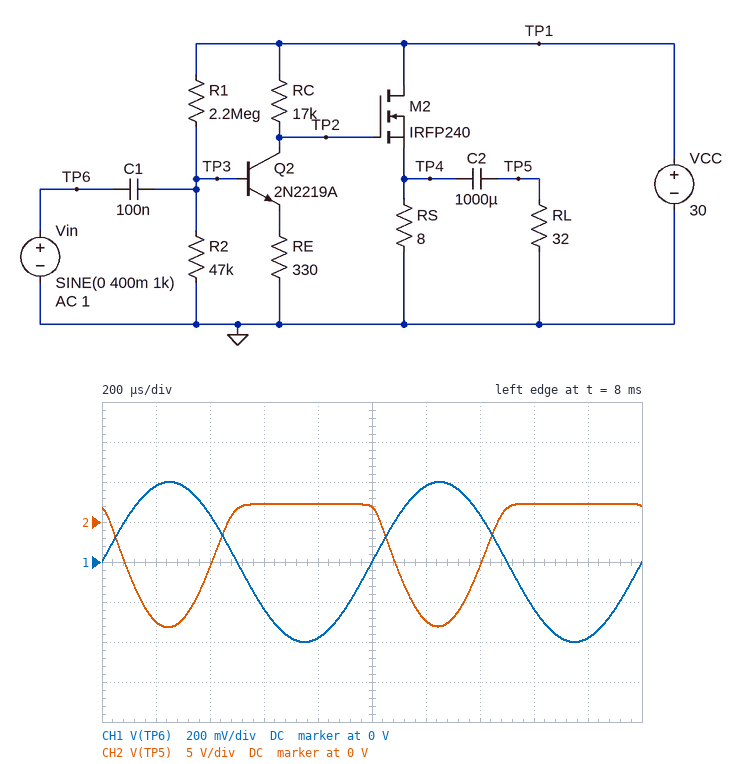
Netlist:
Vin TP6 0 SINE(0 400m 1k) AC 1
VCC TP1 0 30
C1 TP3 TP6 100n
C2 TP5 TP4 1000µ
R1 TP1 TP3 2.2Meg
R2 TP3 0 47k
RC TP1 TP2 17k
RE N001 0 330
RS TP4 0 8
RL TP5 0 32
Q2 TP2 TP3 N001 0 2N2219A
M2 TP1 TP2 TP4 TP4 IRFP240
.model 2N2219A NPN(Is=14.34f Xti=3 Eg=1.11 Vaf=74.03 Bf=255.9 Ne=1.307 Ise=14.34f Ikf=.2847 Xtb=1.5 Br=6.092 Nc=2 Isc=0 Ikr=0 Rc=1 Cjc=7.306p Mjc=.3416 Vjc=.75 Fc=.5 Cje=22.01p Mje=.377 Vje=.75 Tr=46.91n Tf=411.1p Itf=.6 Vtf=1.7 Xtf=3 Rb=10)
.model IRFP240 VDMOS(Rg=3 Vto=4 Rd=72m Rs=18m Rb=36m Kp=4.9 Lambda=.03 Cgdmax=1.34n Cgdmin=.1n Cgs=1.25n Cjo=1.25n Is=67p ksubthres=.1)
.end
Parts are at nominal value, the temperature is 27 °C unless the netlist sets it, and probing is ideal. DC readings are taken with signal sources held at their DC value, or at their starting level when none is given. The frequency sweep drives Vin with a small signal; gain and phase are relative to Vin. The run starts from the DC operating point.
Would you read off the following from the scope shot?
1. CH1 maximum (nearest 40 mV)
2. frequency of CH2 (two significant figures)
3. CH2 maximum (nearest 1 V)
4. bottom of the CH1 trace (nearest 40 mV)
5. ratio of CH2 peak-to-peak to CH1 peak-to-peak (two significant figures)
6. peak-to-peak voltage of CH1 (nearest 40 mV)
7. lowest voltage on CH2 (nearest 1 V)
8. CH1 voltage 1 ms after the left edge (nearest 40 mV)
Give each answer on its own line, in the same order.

400 mV
1.0 kHz
2 V
-400 mV
19
800 mV
-13 V
0 V
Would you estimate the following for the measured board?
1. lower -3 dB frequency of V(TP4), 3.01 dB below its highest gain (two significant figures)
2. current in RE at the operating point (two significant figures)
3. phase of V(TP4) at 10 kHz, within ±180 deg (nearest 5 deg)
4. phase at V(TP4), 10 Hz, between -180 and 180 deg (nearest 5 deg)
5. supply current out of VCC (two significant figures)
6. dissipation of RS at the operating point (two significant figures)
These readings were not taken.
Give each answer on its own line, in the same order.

49 Hz
84 µA
155 deg
-100 deg
2.9 A
69 W
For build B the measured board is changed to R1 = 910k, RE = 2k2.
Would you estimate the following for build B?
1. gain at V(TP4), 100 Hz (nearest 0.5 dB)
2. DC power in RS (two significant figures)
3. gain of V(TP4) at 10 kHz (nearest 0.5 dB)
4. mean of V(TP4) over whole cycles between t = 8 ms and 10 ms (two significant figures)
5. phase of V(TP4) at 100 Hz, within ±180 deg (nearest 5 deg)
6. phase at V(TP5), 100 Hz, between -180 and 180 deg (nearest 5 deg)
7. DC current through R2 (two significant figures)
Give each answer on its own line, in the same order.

16.5 dB
46 W
17.0 dB
19 V
-160 deg
-155 deg
29 µA
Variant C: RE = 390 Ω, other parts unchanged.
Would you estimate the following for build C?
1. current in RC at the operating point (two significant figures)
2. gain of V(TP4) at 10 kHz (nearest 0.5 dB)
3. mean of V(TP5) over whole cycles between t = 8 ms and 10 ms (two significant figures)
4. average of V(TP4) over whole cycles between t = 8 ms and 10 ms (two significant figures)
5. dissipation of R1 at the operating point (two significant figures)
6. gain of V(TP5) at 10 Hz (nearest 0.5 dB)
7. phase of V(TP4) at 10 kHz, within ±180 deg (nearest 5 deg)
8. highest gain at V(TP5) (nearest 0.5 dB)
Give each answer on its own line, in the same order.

79 µA
26.0 dB
-2.1 V
21 V
390 µW
12.5 dB
150 deg
27.0 dB
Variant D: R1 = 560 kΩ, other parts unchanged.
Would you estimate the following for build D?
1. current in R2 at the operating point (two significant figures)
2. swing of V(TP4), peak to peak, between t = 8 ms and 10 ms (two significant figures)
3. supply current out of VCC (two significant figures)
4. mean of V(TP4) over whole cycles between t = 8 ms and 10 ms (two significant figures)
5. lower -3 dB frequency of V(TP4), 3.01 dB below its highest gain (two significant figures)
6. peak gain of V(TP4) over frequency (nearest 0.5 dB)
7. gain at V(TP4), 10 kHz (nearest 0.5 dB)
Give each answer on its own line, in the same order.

26 µA
23 V
1.8 mA
10 V
29 MHz
-15.0 dB
-56.5 dB
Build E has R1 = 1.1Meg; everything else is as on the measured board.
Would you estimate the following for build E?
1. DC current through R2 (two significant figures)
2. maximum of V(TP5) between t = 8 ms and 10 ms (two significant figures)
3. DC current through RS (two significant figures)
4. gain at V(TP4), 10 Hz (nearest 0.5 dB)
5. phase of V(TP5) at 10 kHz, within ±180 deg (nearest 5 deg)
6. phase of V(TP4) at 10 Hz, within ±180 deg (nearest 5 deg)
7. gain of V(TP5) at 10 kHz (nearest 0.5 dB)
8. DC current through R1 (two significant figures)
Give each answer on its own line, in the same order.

21 µA
15 V
1.1 A
17.0 dB
170 deg
-100 deg
33.0 dB
26 µA
